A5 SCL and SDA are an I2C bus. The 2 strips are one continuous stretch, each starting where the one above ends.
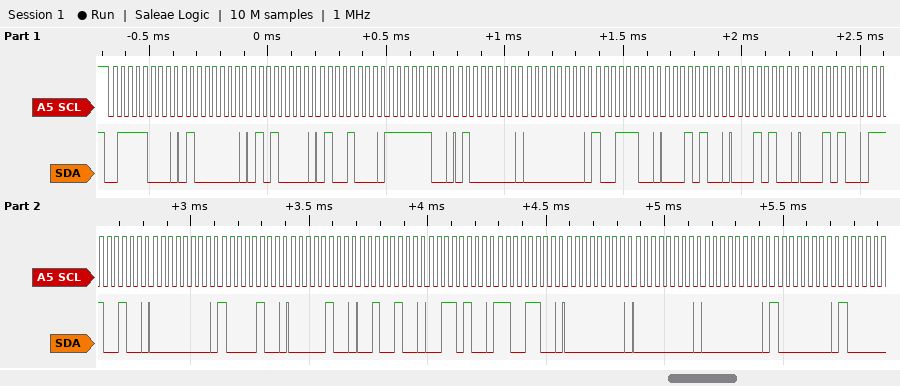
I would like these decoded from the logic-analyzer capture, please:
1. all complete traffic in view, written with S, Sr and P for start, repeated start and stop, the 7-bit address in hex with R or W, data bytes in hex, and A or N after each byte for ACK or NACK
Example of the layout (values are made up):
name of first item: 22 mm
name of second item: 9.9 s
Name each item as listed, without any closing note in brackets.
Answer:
all complete traffic in view, written with S, Sr and P for start, repeated start and stop, the 7-bit address in hex with R or W, data bytes in hex, and A or N after each byte for ACK or NACK: S 3CW A 40 A 50 A 48 A FC A 40 A 00 A 9C A 14 A 14 A 14 A E4 A 00 A 84 A 04 A 24 A 34 A CC A 00 A 00 A 00 A 80 A
